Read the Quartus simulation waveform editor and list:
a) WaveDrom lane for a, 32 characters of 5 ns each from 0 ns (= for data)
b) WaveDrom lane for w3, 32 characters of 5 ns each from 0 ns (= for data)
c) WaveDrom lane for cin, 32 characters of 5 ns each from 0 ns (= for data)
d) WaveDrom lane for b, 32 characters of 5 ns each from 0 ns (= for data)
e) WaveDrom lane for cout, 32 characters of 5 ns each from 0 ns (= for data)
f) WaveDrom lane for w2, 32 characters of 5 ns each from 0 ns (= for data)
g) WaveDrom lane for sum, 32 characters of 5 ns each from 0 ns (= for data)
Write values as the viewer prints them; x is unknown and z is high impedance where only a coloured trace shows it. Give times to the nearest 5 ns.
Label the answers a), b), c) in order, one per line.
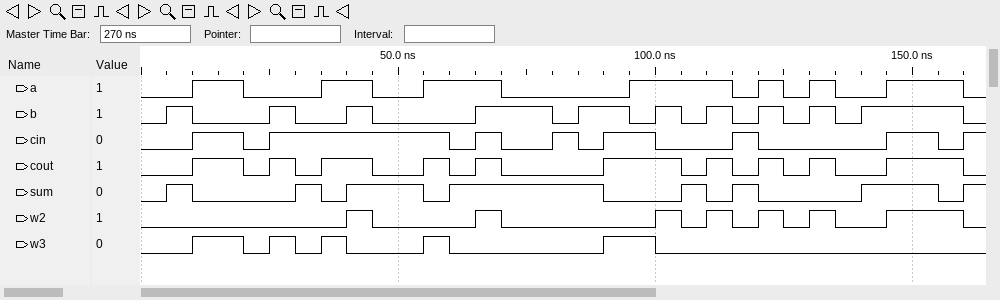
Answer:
a) {name: 'a', wave: '0.1.0..1.0.1..0....1...01010.1..'}
b) {name: 'w3', wave: '0.1.01010..10.....1.0...........'}
c) {name: 'cin', wave: '0.1.01......010.101.0..10....1.0'}
d) {name: 'b', wave: '010..10.10...1..01.0101010101...'}
e) {name: 'cout', wave: '0.1.0101.0.1010...1..0101010.1..'}
f) {name: 'w2', wave: '0.......10...10.....10101010.1..'}
g) {name: 'sum', wave: '010...101..01.....0..1010...1..0'}
